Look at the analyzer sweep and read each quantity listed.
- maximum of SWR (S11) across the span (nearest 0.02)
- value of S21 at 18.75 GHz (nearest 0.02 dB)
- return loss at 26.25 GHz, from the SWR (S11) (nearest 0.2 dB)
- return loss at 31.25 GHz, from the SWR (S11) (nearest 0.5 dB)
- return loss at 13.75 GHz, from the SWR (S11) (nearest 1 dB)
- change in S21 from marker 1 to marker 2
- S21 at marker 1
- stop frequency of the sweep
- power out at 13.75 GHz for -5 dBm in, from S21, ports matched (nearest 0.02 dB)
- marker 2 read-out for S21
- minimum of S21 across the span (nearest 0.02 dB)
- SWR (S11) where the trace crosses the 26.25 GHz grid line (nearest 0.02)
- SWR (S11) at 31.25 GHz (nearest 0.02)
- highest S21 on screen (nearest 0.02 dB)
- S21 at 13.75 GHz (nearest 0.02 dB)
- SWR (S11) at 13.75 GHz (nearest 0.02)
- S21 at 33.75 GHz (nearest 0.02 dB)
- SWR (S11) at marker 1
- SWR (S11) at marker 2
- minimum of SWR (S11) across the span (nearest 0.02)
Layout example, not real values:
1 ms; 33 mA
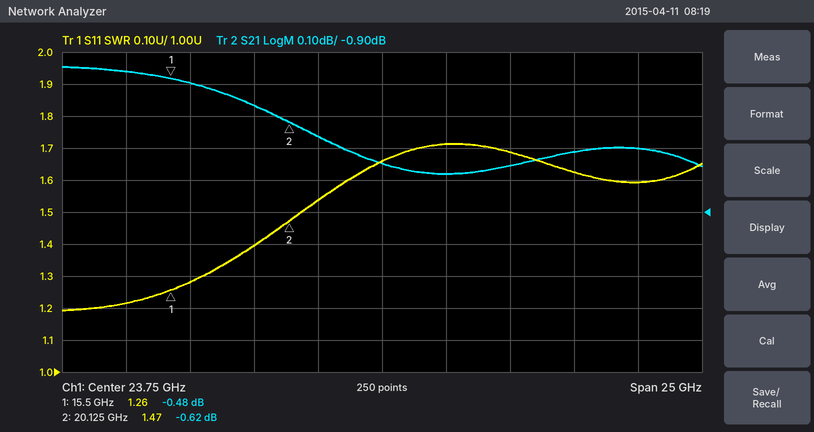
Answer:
1.72; -0.56 dB; 11.6 dB; 12.5 dB; 20 dB; -0.14 dB; -0.48 dB; 36.25 GHz; -5.46 dBm; -0.62 dB; -0.78 dB; 1.72; 1.62; -0.44 dB; -0.46 dB; 1.22; -0.70 dB; 1.26; 1.47; 1.20
